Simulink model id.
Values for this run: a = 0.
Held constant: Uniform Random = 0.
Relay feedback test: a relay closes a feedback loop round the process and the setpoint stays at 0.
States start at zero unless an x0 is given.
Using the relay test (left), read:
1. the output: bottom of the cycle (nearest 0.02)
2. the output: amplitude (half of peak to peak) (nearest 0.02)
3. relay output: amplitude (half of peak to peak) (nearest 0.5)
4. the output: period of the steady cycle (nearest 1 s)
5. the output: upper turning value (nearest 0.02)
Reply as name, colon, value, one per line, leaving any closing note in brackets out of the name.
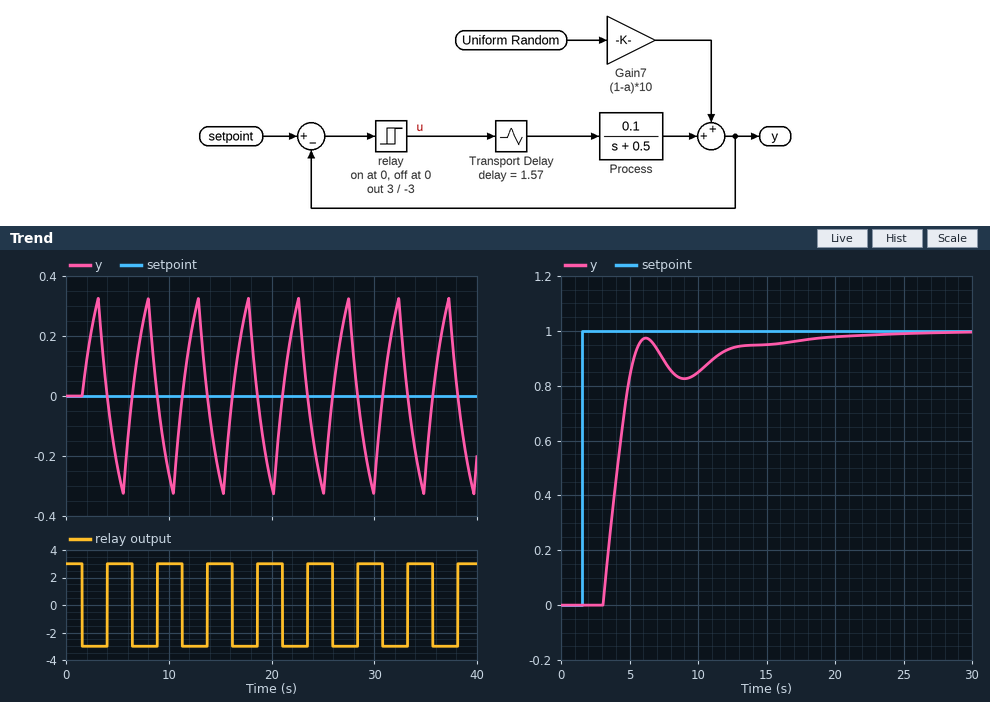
the output: bottom of the cycle: -0.32
the output: amplitude (half of peak to peak): 0.32
relay output: amplitude (half of peak to peak): 3.0
the output: period of the steady cycle: 5 s
the output: upper turning value: 0.32
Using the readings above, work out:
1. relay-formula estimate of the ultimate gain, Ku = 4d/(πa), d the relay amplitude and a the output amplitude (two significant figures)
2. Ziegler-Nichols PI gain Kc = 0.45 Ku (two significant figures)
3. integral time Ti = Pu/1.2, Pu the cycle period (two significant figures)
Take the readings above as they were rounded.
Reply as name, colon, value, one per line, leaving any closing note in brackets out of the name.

relay-formula estimate of the ultimate gain, Ku = 4d/(πa), d the relay amplitude and a the output amplitude: 12
Ziegler-Nichols PI gain Kc = 0.45 Ku: 5.4
integral time Ti = Pu/1.2, Pu the cycle period: 4.2 s
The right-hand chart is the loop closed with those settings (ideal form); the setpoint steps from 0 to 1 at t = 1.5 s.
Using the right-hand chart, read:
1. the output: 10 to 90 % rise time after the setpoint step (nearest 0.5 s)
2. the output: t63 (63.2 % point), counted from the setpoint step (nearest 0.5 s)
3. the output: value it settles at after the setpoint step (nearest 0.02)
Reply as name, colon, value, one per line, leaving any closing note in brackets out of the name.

the output: 10 to 90 % rise time after the setpoint step: 2.0 s
the output: t63 (63.2 % point), counted from the setpoint step: 3.0 s
the output: value it settles at after the setpoint step: 1.00
